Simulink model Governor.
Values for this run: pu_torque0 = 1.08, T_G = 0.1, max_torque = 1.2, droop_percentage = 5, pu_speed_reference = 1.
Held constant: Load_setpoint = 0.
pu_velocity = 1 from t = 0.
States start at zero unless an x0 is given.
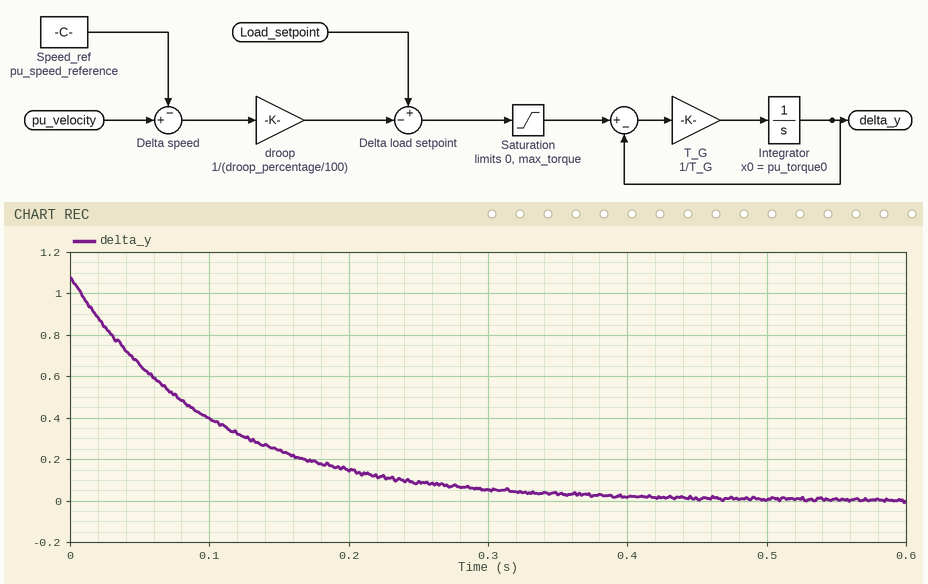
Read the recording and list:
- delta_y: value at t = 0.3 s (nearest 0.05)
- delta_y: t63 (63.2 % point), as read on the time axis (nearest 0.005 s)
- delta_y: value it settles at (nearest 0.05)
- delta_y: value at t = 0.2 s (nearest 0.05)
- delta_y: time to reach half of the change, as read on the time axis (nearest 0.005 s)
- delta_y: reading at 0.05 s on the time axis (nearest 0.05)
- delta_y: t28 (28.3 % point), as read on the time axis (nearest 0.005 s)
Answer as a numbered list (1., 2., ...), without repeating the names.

1. 0.05
2. 0.100 s
3. 0.00
4. 0.15
5. 0.070 s
6. 0.65
7. 0.035 s
